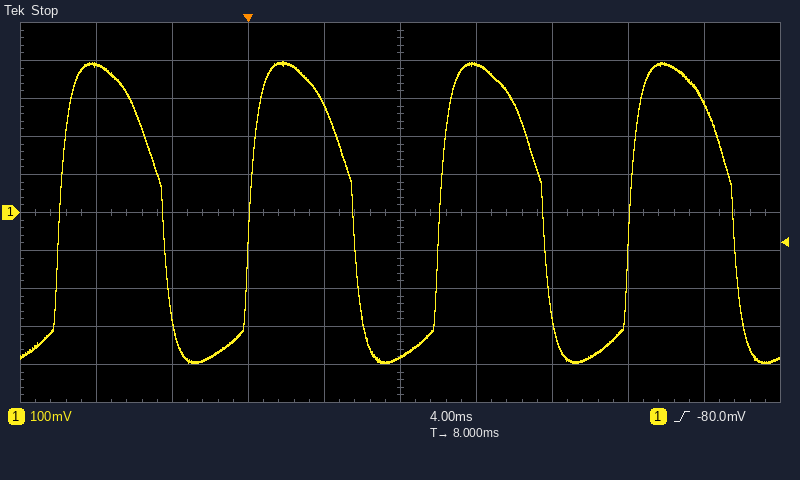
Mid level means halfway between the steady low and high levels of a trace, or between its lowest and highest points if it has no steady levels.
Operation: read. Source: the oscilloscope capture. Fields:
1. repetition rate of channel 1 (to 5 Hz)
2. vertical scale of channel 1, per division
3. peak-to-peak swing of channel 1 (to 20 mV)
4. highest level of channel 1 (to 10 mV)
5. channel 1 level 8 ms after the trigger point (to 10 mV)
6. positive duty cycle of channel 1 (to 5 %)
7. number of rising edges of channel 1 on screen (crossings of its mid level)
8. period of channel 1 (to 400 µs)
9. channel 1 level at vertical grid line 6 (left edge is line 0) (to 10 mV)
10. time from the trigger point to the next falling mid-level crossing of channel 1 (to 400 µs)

100 Hz
100 mV
800 mV
400 mV
-380 mV
55 %
4
10.0 ms
390 mV
5.6 ms
